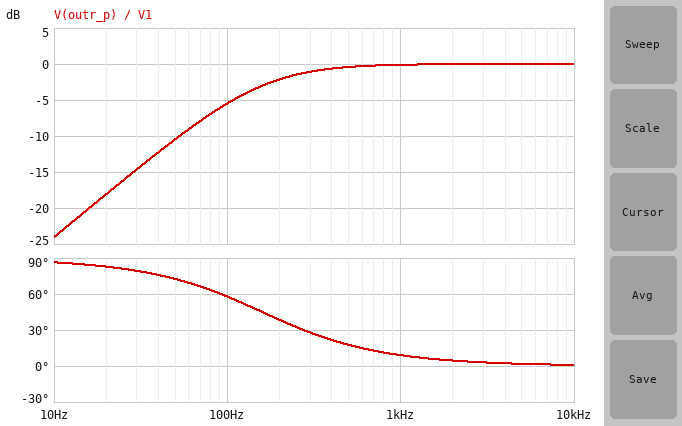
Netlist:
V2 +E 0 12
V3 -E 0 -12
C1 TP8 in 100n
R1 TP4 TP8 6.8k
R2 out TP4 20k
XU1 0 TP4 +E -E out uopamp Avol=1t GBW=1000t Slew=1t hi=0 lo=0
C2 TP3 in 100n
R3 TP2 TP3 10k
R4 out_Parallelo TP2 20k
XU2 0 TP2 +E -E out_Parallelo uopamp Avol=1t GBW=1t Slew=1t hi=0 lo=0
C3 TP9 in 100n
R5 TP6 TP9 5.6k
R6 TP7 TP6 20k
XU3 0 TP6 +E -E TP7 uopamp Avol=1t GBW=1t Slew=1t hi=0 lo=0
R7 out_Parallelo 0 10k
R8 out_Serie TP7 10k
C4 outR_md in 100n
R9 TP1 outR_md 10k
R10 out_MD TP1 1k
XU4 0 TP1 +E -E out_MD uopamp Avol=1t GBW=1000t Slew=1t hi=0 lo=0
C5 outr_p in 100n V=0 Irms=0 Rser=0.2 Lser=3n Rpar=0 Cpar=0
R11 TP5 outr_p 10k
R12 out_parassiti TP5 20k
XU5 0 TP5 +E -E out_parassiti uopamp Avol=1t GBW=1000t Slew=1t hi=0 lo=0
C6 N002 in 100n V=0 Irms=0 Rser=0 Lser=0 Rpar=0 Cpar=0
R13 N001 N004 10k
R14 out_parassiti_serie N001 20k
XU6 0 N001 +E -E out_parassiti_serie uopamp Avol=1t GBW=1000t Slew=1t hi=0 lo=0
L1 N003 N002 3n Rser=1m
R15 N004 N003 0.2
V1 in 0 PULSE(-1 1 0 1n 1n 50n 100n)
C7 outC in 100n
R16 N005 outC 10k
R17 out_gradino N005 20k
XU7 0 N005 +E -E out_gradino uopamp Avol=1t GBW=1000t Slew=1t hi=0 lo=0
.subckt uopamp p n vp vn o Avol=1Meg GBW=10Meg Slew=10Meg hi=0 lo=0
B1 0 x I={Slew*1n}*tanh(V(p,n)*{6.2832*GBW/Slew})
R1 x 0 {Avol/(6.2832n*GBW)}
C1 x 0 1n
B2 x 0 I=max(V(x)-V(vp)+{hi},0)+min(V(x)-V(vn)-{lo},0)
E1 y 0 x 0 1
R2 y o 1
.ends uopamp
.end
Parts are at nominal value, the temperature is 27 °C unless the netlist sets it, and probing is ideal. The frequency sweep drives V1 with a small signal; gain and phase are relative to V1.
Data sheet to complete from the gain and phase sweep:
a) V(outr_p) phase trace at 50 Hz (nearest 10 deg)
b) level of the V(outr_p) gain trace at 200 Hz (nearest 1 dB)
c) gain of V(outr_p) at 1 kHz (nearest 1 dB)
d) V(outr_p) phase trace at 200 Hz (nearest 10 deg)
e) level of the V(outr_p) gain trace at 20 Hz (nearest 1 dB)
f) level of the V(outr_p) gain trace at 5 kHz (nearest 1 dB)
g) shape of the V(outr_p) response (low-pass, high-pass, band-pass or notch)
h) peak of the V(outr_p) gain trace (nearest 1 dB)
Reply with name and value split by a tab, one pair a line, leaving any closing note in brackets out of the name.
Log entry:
V(outr_p) phase trace at 50 Hz	70 deg
level of the V(outr_p) gain trace at 200 Hz	-2 dB
gain of V(outr_p) at 1 kHz	0 dB
V(outr_p) phase trace at 200 Hz	40 deg
level of the V(outr_p) gain trace at 20 Hz	-18 dB
level of the V(outr_p) gain trace at 5 kHz	0 dB
shape of the V(outr_p) response	high-pass
peak of the V(outr_p) gain trace	0 dB
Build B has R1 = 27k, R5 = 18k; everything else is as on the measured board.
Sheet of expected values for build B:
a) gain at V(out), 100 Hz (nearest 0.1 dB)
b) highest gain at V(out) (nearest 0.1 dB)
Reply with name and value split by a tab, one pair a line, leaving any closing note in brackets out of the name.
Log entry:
gain at V(out), 100 Hz	-3.9 dB
highest gain at V(out)	-2.6 dB
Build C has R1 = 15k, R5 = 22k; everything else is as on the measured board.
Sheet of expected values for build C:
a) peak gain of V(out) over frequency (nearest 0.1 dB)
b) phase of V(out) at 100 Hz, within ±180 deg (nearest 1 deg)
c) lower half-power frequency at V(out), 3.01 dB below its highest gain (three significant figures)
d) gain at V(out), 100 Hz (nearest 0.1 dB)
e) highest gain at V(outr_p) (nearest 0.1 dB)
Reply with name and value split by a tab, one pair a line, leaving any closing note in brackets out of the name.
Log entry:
peak gain of V(out) over frequency	2.5 dB
phase of V(out) at 100 Hz, within ±180 deg	-133 deg
lower half-power frequency at V(out), 3.01 dB below its highest gain	106 Hz
gain at V(out), 100 Hz	-0.8 dB
highest gain at V(outr_p)	0 dB
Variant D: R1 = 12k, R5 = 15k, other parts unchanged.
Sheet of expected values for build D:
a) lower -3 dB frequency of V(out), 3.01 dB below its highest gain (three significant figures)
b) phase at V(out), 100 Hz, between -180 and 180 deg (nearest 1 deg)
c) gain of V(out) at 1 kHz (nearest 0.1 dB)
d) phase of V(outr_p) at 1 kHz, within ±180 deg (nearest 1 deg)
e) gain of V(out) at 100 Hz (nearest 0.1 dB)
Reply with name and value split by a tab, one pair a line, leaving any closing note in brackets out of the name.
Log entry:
lower -3 dB frequency of V(out), 3.01 dB below its highest gain	133 Hz
phase at V(out), 100 Hz, between -180 and 180 deg	-127 deg
gain of V(out) at 1 kHz	4.4 dB
phase of V(outr_p) at 1 kHz, within ±180 deg	9 deg
gain of V(out) at 100 Hz	0 dB
